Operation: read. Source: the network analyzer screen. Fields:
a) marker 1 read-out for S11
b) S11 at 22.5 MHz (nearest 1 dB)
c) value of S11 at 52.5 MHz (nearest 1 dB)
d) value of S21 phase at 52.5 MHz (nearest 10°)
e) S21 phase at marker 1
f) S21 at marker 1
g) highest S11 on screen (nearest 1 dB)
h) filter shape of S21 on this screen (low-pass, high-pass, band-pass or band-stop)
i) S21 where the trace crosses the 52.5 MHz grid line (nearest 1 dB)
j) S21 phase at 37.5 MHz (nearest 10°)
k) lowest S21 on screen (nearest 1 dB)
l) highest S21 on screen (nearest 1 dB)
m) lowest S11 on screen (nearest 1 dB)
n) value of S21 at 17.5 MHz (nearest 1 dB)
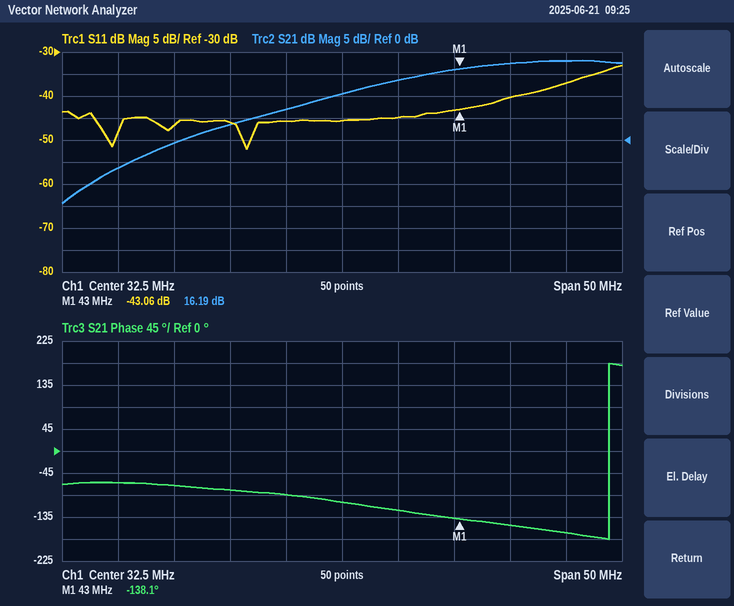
-43.06 dB
-46 dB
-37 dB
-170°
-138.1°
16.19 dB
-33 dB
high-pass
18 dB
-120°
-14 dB
18 dB
-52 dB
-1 dB
